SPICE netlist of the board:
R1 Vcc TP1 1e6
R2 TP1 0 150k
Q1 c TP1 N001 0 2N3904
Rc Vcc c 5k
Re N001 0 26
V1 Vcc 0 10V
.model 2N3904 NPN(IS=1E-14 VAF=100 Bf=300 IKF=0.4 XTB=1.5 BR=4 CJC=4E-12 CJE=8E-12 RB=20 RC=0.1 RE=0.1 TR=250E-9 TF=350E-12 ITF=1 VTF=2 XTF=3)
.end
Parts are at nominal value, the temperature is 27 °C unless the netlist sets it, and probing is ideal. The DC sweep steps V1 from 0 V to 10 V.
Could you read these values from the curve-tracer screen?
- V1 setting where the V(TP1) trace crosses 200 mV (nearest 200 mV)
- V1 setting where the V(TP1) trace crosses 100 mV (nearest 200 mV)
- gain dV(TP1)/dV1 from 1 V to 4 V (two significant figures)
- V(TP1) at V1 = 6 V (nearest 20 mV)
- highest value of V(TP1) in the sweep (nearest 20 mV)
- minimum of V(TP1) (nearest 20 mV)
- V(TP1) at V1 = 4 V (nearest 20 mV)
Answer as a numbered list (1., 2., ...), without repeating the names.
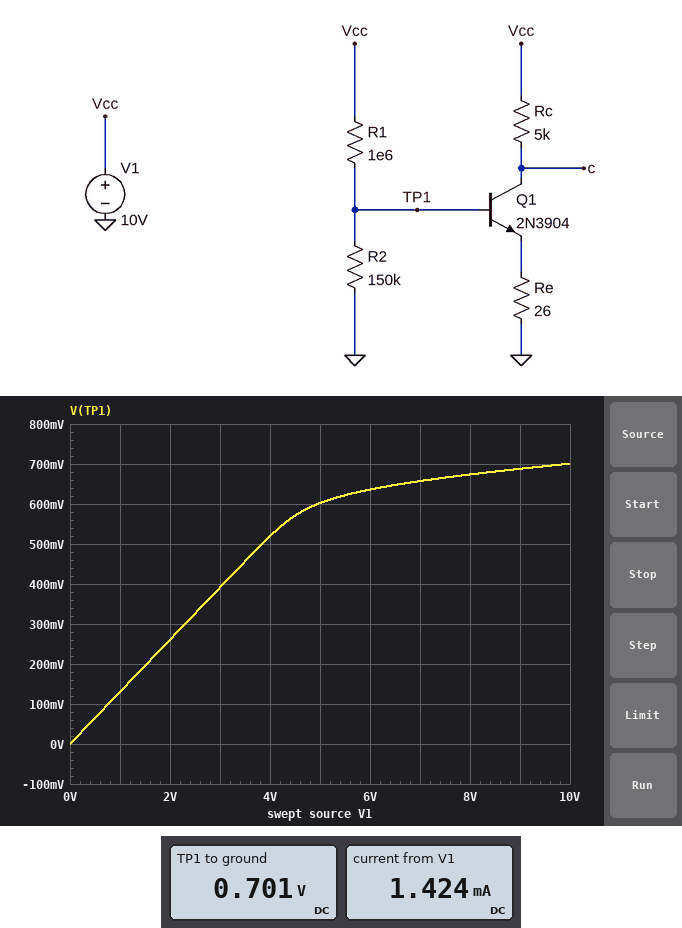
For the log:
1. 1.6 V
2. 800 mV
3. 0.13 V/V
4. 640 mV
5. 700 mV
6. 0 V
7. 520 mV
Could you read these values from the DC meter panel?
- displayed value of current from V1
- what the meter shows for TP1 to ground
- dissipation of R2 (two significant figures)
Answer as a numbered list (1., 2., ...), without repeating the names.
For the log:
1. 1.424 mA
2. 0.701 V
3. 3.3 µW
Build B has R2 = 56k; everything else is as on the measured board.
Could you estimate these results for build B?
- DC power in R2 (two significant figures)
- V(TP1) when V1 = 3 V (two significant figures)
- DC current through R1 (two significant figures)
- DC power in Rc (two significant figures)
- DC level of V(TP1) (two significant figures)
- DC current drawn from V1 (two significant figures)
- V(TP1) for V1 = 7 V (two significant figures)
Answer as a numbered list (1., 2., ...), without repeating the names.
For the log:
1. 5.0 µW
2. 160 mV
3. 9.5 µA
4. 340 nW
5. 530 mV
6. 18 µA
7. 370 mV
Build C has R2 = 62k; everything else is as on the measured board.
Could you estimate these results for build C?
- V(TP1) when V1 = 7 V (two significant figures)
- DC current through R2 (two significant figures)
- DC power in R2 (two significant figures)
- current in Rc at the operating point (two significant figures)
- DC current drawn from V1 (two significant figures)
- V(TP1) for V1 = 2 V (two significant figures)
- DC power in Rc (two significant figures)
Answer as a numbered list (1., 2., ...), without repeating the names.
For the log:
1. 410 mV
2. 9.3 µA
3. 5.3 µW
4. 48 µA
5. 57 µA
6. 120 mV
7. 11 µW
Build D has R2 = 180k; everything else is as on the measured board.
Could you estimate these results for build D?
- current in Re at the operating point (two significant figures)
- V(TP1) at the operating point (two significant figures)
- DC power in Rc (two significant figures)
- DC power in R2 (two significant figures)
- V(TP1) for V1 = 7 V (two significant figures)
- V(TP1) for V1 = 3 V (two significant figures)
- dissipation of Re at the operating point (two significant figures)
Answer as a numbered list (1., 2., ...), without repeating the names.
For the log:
1. 1.6 mA
2. 710 mV
3. 13 mW
4. 2.8 µW
5. 670 mV
6. 460 mV
7. 68 µW
